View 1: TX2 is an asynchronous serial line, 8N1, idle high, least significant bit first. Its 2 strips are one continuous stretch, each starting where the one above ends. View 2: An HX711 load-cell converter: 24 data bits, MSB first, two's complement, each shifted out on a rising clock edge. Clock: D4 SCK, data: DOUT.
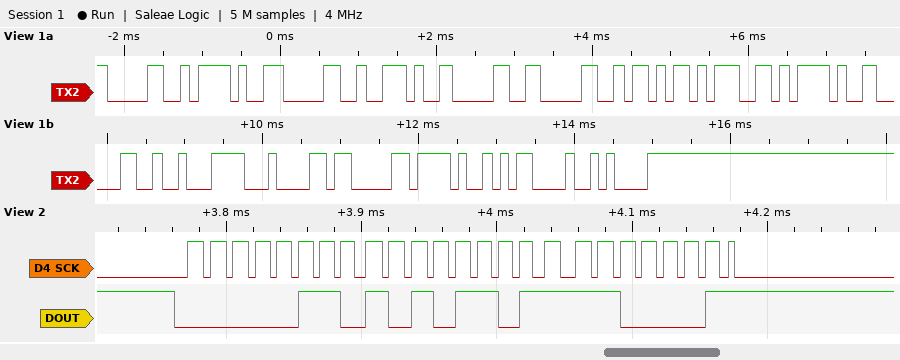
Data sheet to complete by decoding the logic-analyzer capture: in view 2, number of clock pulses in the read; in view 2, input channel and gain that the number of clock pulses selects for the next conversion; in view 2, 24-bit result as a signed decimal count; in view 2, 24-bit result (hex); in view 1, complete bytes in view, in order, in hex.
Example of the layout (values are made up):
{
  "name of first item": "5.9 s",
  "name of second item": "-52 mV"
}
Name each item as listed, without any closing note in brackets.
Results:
{
  "in view 2, number of clock pulses in the read": "25",
  "in view 2, input channel and gain that the number of clock pulses selects for the next conversion": "channel A, gain 128",
  "in view 2, 24-bit result as a signed decimal count": "437729",
  "in view 2, 24-bit result": "0x06ADE1",
  "in view 1, complete bytes in view, in order, in hex": "30 2F 30 2E 30 30 6B 67 2F 30 E2 84 83 2F 0D 0A"
}
